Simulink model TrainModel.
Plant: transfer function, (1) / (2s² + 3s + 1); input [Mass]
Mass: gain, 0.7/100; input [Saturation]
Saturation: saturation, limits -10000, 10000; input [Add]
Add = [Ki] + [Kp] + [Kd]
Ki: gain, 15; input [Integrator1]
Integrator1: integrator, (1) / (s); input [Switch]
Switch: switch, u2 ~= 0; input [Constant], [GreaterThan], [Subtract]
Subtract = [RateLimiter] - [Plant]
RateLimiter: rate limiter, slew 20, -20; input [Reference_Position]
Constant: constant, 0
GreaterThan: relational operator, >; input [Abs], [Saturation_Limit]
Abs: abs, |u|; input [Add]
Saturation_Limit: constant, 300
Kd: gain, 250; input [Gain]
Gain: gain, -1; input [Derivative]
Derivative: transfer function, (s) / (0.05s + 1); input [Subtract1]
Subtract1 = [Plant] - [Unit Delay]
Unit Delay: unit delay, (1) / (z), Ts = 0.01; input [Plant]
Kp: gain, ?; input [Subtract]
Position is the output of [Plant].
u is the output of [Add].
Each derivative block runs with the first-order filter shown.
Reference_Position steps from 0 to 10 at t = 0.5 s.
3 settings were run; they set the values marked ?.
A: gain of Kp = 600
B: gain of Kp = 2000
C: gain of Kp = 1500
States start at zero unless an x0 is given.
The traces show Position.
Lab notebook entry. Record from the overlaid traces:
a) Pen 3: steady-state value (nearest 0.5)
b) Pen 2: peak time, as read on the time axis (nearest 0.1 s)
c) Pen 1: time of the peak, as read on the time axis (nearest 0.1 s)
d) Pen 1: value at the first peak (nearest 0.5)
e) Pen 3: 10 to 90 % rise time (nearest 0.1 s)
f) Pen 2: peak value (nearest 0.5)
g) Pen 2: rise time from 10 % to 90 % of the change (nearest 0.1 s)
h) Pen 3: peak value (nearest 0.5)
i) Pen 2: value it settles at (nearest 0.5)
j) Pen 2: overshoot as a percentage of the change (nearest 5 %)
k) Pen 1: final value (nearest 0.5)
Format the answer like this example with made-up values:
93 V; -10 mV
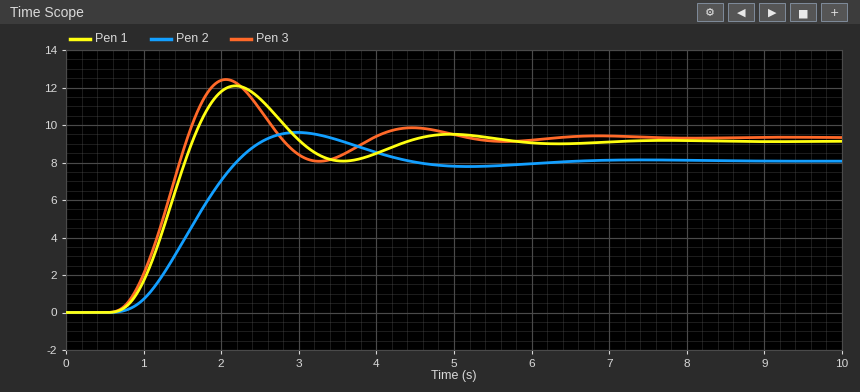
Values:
9.5; 3.0 s; 2.2 s; 12.0; 0.6 s; 9.5; 1.0 s; 12.5; 8.0; 20 %; 9.0
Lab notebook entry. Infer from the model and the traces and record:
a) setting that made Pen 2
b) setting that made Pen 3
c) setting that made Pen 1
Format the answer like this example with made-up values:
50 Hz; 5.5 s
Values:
A; B; C
